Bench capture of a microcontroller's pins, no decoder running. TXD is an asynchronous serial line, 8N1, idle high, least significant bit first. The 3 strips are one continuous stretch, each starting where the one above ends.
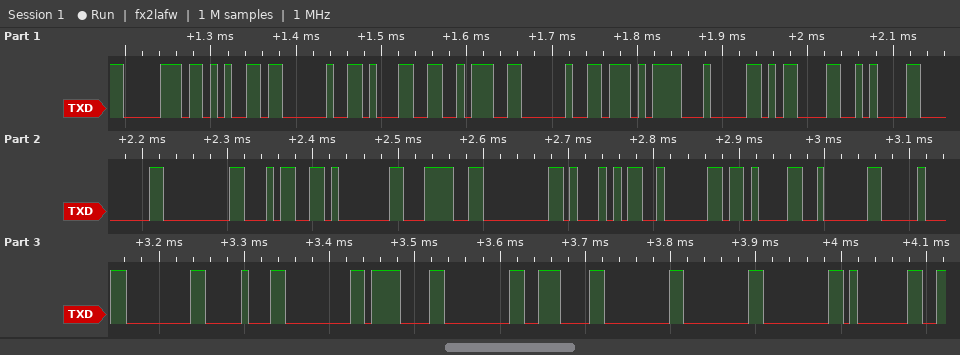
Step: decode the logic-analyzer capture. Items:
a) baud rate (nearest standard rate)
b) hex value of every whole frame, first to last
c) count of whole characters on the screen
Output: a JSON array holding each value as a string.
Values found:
["115200 baud", "0x70 0x65 0x20 0x31 0x3A 0x20 0xD7 0x04 0x0D 0x0A 0x00 0x00 0x34 0x01 0x3C 0x00 0x51 0x02 0x0B 0x02 0x10 0x00 0x10 0x00 0x0F 0x00 0x0E 0x00 0x00 0x00 0x01", "31"]
